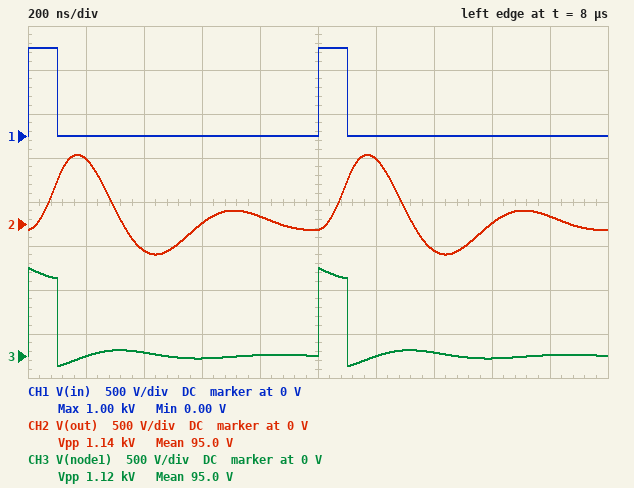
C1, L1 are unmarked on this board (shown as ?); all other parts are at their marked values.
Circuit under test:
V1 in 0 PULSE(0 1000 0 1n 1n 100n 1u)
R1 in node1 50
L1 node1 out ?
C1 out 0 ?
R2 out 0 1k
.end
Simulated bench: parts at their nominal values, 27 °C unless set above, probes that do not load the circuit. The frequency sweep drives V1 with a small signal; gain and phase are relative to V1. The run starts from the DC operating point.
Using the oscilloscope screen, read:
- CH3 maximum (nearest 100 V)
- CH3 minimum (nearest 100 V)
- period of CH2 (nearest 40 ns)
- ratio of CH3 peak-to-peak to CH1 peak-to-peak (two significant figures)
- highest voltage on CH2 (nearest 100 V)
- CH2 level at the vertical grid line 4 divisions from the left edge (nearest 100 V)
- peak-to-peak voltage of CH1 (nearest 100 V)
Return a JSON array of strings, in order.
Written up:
["1.0 kV", "-100 V", "1.00 µs", "1.1", "800 V", "100 V", "1.0 kV"]
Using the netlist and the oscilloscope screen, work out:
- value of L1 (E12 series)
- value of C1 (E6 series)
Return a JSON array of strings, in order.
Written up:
["33 µH", "220 pF"]
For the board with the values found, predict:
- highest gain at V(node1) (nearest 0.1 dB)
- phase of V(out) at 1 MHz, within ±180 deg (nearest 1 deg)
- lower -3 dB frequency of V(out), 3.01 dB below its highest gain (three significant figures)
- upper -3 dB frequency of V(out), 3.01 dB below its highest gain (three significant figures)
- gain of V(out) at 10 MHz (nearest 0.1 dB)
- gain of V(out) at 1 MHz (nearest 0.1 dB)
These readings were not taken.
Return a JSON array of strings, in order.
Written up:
["0 dB", "-20 deg", "1.19 MHz", "2.23 MHz", "-28.9 dB", "1.8 dB"]
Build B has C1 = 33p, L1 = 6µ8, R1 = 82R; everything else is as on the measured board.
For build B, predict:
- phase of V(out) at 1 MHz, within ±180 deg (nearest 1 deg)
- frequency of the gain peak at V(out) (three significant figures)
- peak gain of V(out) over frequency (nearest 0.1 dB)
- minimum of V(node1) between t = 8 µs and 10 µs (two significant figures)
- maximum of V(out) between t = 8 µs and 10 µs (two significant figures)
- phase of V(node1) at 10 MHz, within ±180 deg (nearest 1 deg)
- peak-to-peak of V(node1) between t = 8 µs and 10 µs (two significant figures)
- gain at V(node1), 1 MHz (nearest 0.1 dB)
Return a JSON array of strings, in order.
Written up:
["-3 deg", "9.97 MHz", "4.0 dB", "-69 V", "1.3 kV", "3 deg", "1.1 kV", "-0.7 dB"]
